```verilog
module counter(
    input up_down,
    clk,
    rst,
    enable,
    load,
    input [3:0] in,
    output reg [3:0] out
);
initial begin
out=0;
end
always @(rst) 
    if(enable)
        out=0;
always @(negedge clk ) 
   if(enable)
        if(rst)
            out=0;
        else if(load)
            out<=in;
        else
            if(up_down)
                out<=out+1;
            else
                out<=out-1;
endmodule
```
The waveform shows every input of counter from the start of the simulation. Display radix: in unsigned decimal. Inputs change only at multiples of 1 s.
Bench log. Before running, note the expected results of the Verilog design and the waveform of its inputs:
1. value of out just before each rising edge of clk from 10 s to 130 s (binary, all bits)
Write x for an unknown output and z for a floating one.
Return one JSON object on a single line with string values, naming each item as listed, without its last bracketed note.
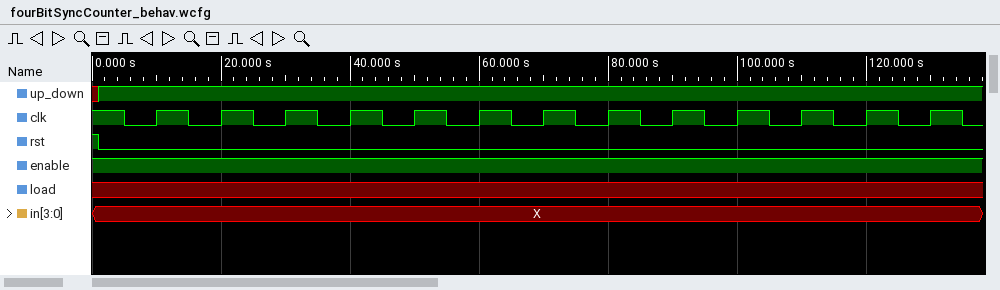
{"value of out just before each rising edge of clk from 10 s to 130 s": "0001, 0010, 0011, 0100, 0101, 0110, 0111, 1000, 1001, 1010, 1011, 1100, 1101"}
